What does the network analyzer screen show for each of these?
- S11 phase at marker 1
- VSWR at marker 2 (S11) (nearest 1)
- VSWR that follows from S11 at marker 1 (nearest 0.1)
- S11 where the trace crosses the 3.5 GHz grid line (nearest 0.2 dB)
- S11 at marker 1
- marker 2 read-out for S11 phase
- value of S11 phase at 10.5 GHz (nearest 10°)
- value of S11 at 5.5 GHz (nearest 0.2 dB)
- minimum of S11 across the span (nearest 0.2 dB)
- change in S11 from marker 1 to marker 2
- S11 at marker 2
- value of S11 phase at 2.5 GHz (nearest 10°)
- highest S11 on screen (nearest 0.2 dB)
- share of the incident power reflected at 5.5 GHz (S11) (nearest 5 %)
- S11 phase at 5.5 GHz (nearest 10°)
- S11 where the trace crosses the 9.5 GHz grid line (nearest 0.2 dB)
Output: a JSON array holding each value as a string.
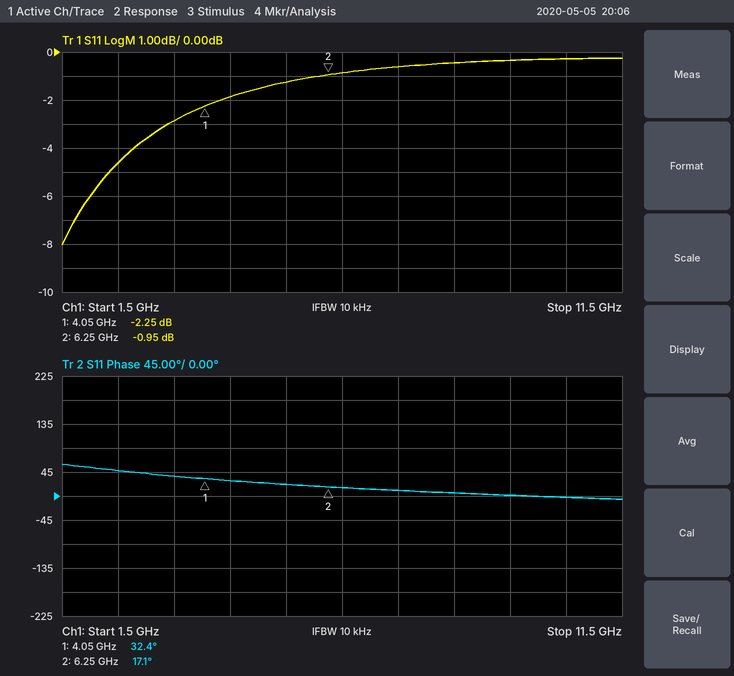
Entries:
["32.4°", "18", "7.8", "-2.8 dB", "-2.25 dB", "17.1°", "0°", "-1.2 dB", "-8.0 dB", "1.30 dB", "-0.95 dB", "50°", "-0.2 dB", "75 %", "20°", "-0.4 dB"]
